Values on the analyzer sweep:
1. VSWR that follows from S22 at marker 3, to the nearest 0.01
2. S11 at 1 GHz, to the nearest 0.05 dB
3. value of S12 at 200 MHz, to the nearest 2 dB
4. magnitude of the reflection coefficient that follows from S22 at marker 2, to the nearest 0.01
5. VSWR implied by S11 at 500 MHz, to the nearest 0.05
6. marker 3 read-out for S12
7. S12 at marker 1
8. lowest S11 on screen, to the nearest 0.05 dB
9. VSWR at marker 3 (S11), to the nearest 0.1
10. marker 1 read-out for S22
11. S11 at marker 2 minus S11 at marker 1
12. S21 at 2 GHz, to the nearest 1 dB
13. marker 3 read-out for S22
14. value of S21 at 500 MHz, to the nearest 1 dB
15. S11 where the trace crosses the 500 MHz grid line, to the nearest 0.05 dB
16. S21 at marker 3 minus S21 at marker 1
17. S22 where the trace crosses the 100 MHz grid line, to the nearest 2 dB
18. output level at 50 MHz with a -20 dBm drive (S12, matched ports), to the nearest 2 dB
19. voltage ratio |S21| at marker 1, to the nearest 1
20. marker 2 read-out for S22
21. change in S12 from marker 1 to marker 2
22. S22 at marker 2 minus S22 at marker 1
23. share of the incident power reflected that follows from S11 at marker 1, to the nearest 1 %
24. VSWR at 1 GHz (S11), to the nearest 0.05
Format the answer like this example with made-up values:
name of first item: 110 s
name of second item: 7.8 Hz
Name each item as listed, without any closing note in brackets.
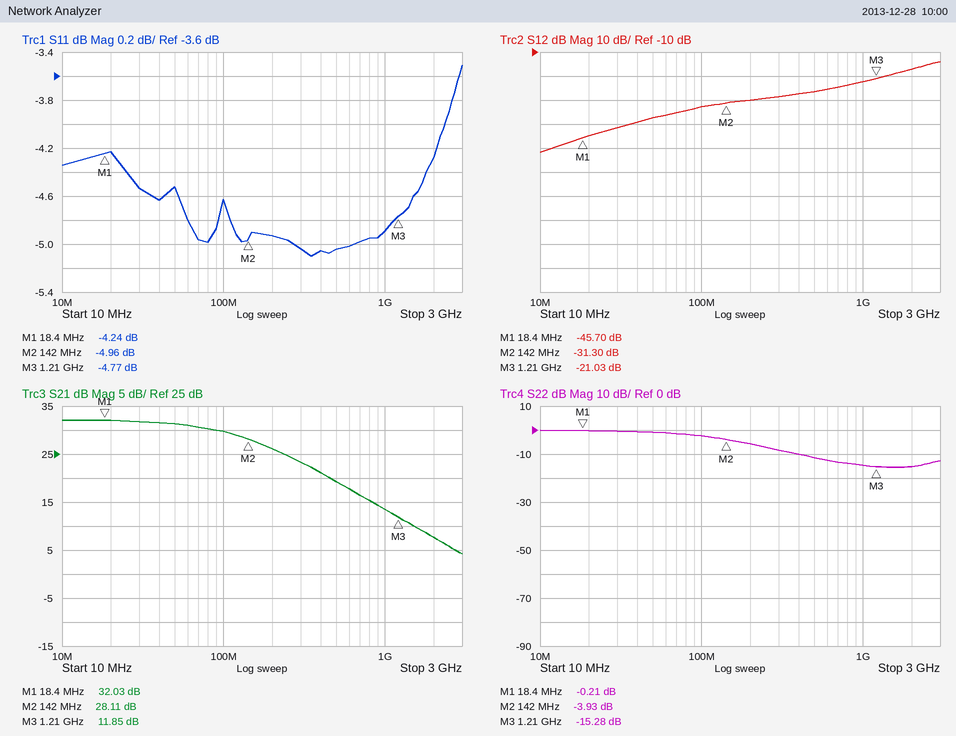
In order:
VSWR that follows from S22 at marker 3, to the nearest 0.01: 1.42
S11 at 1 GHz, to the nearest 0.05 dB: -4.90 dB
value of S12 at 200 MHz, to the nearest 2 dB: -30 dB
magnitude of the reflection coefficient that follows from S22 at marker 2, to the nearest 0.01: 0.64
VSWR implied by S11 at 500 MHz, to the nearest 0.05: 3.55
marker 3 read-out for S12: -21.03 dB
S12 at marker 1: -45.70 dB
lowest S11 on screen, to the nearest 0.05 dB: -5.10 dB
VSWR at marker 3 (S11), to the nearest 0.1: 3.7
marker 1 read-out for S22: -0.21 dB
S11 at marker 2 minus S11 at marker 1: -0.72 dB
S21 at 2 GHz, to the nearest 1 dB: 8 dB
marker 3 read-out for S22: -15.28 dB
value of S21 at 500 MHz, to the nearest 1 dB: 19 dB
S11 where the trace crosses the 500 MHz grid line, to the nearest 0.05 dB: -5.05 dB
S21 at marker 3 minus S21 at marker 1: -20.18 dB
S22 where the trace crosses the 100 MHz grid line, to the nearest 2 dB: -2 dB
output level at 50 MHz with a -20 dBm drive (S12, matched ports), to the nearest 2 dB: -58 dBm
voltage ratio |S21| at marker 1, to the nearest 1: 40
marker 2 read-out for S22: -3.93 dB
change in S12 from marker 1 to marker 2: 14.40 dB
S22 at marker 2 minus S22 at marker 1: -3.72 dB
share of the incident power reflected that follows from S11 at marker 1, to the nearest 1 %: 38 %
VSWR at 1 GHz (S11), to the nearest 0.05: 3.65
